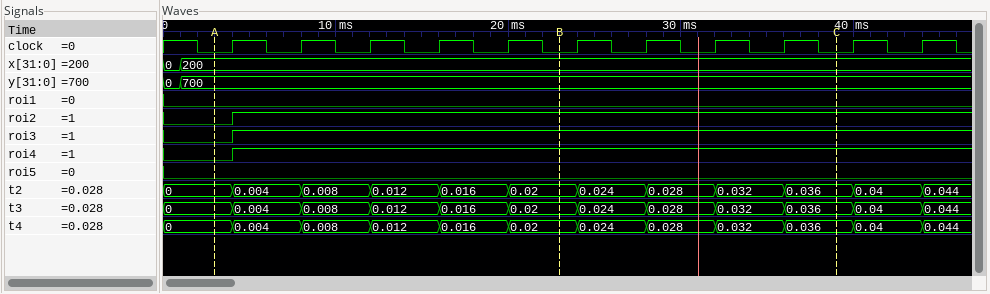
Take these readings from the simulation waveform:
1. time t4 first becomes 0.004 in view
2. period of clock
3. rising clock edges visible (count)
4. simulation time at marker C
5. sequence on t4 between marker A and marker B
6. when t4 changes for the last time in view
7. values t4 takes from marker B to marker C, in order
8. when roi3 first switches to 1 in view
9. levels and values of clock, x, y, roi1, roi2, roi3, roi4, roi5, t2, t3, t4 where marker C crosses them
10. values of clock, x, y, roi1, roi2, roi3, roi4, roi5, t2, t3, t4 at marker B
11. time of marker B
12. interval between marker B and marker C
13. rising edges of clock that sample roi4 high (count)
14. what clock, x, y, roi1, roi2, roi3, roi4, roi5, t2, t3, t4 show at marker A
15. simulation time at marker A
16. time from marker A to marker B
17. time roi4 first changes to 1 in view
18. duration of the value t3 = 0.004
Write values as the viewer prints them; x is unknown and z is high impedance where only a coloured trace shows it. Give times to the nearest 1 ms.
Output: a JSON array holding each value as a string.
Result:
["4 ms", "4 ms", "11", "39 ms", "0, 0.004, 0.008, 0.012, 0.016, 0.02", "44 ms", "0.02, 0.024, 0.028, 0.032, 0.036", "4 ms", "clock=0, x=200, y=700, roi1=0, roi2=1, roi3=1, roi4=1, roi5=0, t2=0.036, t3=0.036, t4=0.036", "clock=0, x=200, y=700, roi1=0, roi2=1, roi3=1, roi4=1, roi5=0, t2=0.02, t3=0.02, t4=0.02", "23 ms", "16 ms", "10", "clock=0, x=200, y=700, roi1=0, roi2=0, roi3=0, roi4=0, roi5=0, t2=0, t3=0, t4=0", "3 ms", "20 ms", "4 ms", "4 ms"]
